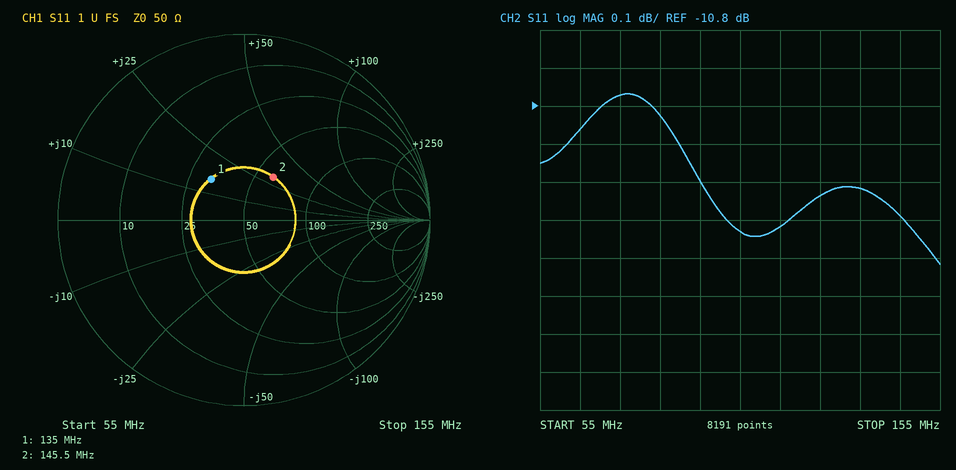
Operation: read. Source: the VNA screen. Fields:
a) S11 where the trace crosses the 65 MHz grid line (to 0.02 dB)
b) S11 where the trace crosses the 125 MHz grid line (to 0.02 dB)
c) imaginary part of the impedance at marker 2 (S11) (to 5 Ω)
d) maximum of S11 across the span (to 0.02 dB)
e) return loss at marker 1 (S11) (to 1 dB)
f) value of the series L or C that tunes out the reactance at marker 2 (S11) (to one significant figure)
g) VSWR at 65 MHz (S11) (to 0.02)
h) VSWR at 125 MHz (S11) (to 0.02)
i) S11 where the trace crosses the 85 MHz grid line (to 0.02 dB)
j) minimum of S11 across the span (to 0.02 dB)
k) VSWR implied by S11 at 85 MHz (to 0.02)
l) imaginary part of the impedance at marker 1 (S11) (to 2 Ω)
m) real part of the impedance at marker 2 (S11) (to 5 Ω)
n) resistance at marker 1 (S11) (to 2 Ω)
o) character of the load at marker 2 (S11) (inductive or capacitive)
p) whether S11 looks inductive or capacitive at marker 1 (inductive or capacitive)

-10.86 dB
-11.04 dB
+30 Ω
-10.76 dB
11 dB
40 pF
1.80
1.78
-10.82 dB
-11.22 dB
1.80
+16 Ω
60 Ω
32 Ω
inductive
inductive
